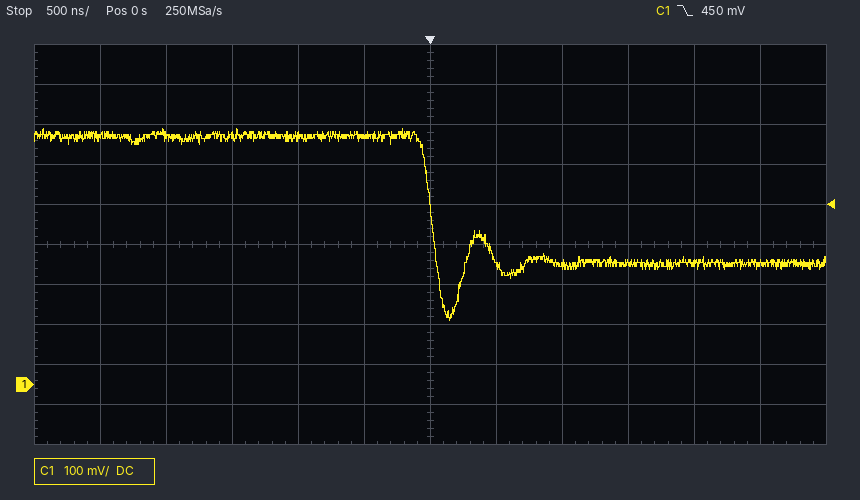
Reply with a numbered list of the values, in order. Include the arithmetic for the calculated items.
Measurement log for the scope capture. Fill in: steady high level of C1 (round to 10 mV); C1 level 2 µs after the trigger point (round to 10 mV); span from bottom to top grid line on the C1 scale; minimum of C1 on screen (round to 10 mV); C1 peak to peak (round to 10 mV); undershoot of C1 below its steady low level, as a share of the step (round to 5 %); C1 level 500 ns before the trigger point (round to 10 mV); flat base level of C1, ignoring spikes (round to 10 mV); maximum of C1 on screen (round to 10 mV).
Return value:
1. 620 mV
2. 300 mV
3. 1 V
4. 160 mV
5. 640 mV − (160 mV) = 480 mV
6. 45 %
7. 620 mV
8. 300 mV
9. 640 mV
